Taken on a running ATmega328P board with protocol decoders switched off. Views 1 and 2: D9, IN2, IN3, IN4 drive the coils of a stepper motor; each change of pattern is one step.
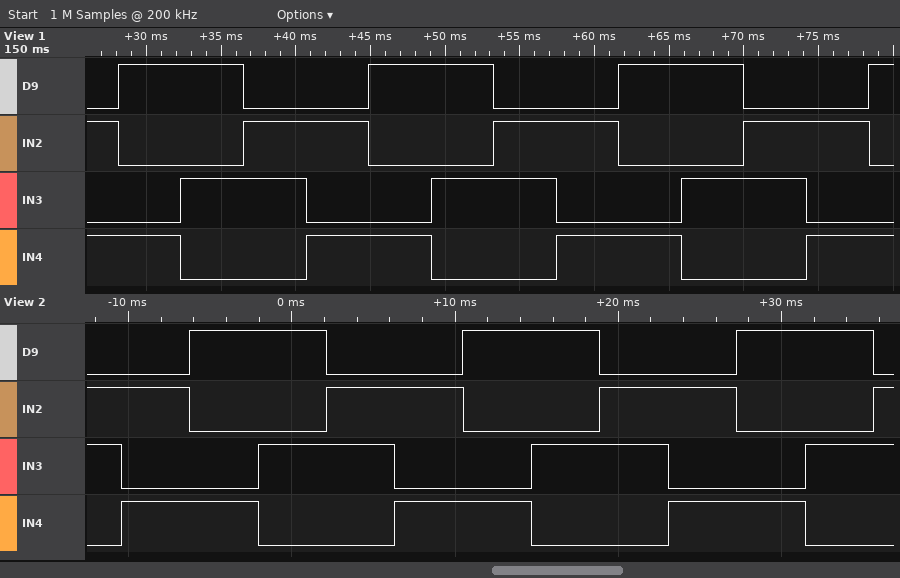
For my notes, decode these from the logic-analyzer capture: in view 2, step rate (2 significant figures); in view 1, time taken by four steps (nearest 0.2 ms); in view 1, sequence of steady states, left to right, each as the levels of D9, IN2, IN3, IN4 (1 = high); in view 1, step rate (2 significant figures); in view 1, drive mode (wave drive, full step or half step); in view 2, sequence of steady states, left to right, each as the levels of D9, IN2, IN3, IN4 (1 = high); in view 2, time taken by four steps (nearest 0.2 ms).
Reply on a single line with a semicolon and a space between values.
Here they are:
240 steps/s; 16.8 ms; 0101 1001 1010 0110 0101 1001 1010 0110 0101 1001 1010 0110 0101 1001; 240 steps/s; full step; 0110 0101 1001 1010 0110 0101 1001 1010 0110 0101 1001 1010 0110; 16.8 ms
